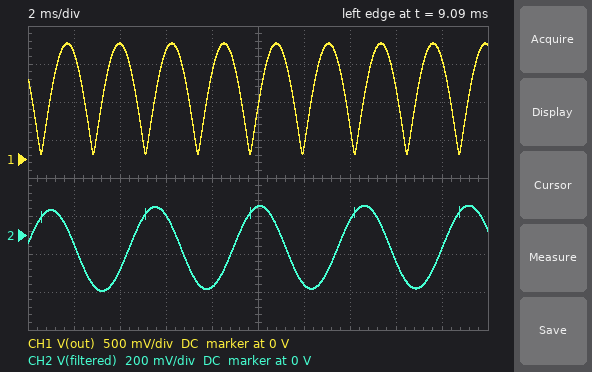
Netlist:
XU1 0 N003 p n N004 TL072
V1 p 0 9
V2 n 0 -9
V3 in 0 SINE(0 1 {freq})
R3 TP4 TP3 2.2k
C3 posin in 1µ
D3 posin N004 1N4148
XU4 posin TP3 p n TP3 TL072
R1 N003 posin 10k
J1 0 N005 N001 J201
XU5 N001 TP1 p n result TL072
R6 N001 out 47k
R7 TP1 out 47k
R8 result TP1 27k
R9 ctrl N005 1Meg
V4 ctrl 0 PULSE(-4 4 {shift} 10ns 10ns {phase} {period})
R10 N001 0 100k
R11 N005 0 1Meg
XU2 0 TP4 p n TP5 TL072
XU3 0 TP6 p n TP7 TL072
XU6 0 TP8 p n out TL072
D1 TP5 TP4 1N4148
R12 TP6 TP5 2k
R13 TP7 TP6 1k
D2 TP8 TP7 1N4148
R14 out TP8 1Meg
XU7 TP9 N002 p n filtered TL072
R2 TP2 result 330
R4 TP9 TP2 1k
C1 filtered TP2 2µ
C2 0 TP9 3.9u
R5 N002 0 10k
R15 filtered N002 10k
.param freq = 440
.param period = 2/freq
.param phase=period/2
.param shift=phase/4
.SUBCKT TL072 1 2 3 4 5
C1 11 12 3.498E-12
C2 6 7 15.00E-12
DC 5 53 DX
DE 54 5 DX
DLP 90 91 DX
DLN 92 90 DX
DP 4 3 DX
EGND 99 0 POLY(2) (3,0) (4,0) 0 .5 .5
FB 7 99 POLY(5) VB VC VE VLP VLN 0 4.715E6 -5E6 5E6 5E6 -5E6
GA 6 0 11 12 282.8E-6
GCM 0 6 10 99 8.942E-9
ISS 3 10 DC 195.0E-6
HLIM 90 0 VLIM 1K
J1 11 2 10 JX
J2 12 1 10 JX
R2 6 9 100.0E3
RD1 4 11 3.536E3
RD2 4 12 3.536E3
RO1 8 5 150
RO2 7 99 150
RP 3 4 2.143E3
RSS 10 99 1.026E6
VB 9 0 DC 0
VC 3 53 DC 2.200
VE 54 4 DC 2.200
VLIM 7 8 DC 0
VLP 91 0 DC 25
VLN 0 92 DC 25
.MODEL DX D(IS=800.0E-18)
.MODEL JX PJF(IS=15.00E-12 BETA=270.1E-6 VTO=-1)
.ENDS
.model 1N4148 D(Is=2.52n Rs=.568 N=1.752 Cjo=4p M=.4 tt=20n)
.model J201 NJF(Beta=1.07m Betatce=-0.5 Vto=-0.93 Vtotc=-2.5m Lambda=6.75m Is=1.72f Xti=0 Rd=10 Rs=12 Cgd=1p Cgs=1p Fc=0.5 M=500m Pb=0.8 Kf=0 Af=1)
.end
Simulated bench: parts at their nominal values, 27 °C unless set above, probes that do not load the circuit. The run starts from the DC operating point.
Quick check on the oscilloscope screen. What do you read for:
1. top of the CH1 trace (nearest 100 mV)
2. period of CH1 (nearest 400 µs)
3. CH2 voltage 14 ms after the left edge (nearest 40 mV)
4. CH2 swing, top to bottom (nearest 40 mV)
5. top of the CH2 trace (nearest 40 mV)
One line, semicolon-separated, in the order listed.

1.5 V; 2.4 ms; 80 mV; 440 mV; 160 mV
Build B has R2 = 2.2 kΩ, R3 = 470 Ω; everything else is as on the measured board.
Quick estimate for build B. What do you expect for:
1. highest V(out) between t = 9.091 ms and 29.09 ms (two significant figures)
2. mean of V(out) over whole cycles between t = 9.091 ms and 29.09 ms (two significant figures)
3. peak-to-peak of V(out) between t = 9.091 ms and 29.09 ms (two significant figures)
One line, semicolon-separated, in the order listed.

3.4 V; 2.1 V; 3.2 V
